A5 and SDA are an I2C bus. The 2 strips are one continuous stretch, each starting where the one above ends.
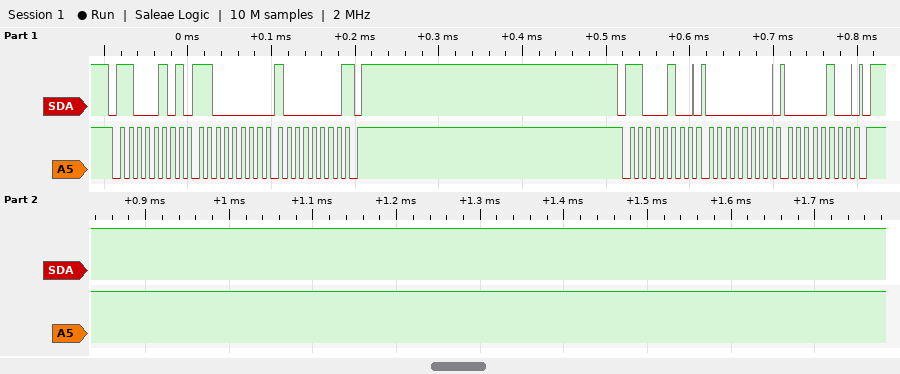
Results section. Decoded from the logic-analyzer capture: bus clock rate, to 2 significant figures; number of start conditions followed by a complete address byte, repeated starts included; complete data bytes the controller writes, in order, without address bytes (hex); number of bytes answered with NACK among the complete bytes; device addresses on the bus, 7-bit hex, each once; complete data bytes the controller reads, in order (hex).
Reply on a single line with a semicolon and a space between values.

100 kHz; 2; 00 04; 1; 0x62; C0 80
